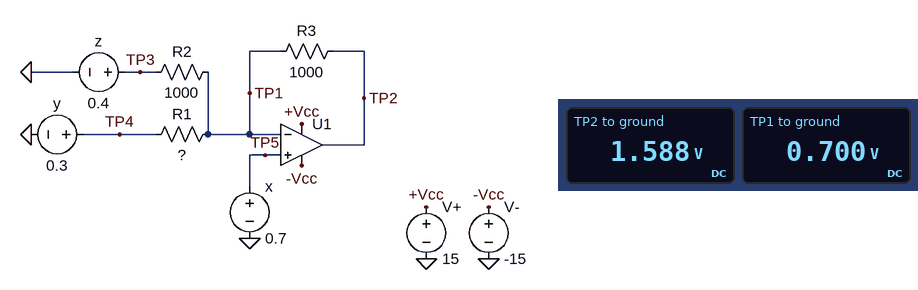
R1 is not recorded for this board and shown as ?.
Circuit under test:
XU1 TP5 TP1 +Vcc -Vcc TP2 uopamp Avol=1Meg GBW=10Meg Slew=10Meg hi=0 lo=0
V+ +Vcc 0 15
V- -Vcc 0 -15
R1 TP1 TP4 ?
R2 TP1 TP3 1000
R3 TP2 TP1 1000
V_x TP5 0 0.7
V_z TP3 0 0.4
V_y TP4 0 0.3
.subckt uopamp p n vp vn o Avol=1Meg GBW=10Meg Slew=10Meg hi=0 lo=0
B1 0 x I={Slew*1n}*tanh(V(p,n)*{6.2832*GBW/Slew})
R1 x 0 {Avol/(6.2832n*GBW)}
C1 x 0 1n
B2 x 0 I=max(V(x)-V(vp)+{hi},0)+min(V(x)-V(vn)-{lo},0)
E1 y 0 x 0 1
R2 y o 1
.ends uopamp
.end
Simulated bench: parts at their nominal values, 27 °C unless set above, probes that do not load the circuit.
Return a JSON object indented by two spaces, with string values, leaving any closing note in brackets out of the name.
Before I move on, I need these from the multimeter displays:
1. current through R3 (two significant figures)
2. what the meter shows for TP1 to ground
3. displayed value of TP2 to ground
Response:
{
  "current through R3": "890 µA",
  "what the meter shows for TP1 to ground": "0.700 V",
  "displayed value of TP2 to ground": "1.588 V"
}
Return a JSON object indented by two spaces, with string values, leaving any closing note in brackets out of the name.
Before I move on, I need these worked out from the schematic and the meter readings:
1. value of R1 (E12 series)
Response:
{
  "value of R1": "680 Ω"
}
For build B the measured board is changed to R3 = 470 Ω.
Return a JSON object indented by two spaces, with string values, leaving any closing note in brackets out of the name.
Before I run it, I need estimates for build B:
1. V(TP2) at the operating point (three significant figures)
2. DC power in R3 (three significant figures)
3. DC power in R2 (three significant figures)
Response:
{
  "V(TP2) at the operating point": "1.12 V",
  "DC power in R3": "371 µW",
  "DC power in R2": "90.0 µW"
}
